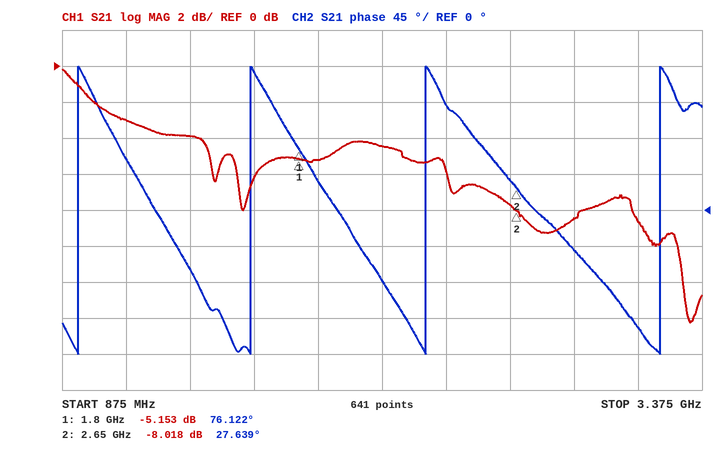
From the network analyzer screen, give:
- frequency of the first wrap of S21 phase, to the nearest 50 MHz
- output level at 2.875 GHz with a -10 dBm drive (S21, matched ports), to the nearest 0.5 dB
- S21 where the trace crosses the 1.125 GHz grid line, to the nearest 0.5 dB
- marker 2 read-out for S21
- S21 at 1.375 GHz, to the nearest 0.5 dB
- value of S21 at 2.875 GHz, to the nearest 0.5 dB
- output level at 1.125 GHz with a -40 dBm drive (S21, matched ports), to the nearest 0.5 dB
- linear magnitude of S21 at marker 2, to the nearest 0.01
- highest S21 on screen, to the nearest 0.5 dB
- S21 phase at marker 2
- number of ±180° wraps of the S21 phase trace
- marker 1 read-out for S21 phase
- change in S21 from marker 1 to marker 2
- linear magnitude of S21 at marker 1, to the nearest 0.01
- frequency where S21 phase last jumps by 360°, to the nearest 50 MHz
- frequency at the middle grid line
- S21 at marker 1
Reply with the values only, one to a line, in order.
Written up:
950 MHz
-18.5 dBm
-3.0 dB
-8.018 dB
-4.0 dB
-8.5 dB
-43.0 dBm
0.40
0.0 dB
27.639°
4
76.122°
-2.865 dB
0.55
3.20 GHz
2.125 GHz
-5.153 dB
